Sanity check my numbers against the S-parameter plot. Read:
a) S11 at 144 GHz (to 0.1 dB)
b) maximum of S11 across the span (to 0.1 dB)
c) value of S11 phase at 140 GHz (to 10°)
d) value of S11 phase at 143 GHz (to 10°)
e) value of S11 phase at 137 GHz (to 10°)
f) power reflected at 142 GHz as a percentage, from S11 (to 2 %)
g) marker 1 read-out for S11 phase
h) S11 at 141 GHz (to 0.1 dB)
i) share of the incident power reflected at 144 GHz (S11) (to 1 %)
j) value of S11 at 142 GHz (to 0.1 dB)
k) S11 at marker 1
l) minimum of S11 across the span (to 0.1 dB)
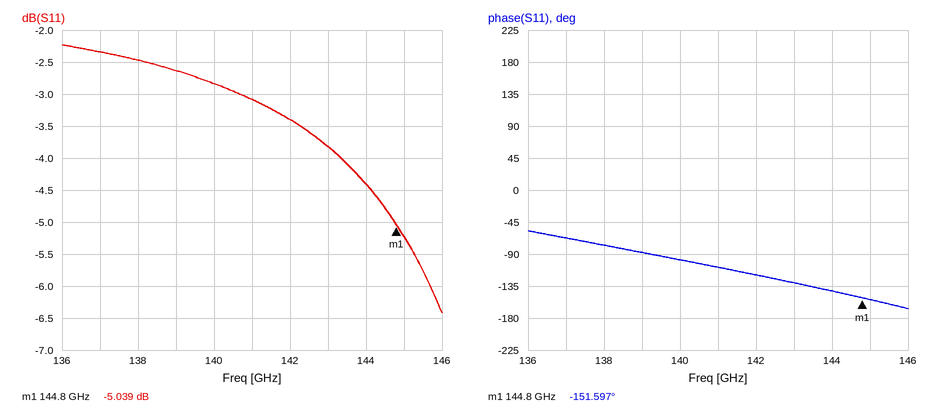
-4.4 dB
-2.2 dB
-100°
-130°
-70°
46 %
-151.597°
-3.1 dB
36 %
-3.4 dB
-5.039 dB
-6.4 dB
